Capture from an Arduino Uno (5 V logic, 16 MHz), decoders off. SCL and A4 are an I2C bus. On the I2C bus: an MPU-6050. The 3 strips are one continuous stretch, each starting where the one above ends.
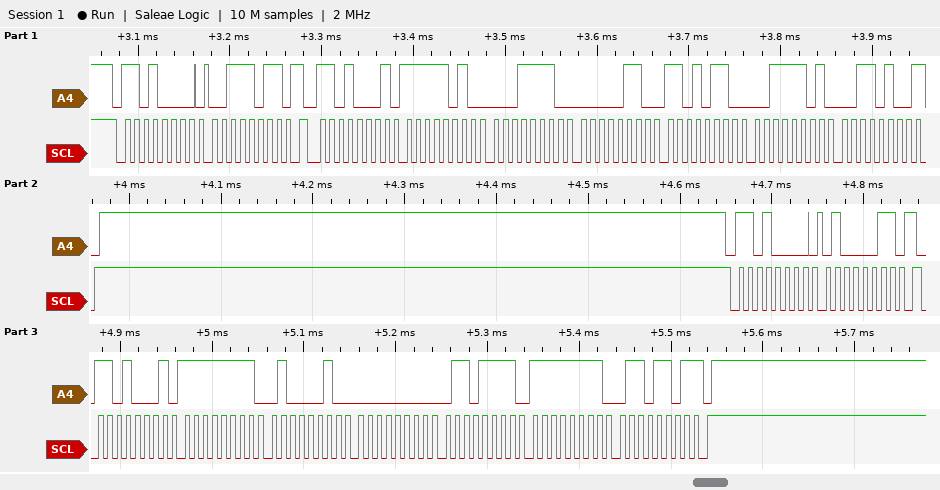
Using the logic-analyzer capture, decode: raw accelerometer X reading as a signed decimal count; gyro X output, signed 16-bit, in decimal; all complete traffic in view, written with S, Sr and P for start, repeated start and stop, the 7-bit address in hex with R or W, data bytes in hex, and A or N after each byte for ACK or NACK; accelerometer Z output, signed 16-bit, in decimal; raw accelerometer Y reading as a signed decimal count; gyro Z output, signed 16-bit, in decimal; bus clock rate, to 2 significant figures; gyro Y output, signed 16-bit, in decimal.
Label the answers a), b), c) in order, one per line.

a) -1506
b) -190
c) S 68W A 3B A Sr 68R A FA A 1E A 06 A D6 A 3D A 34 N P S 68W A 43 A Sr 68R A FF A 42 A 00 A 6F A FF A 6D N P
d) 15668
e) 1750
f) -147
g) 100 kHz
h) 111
